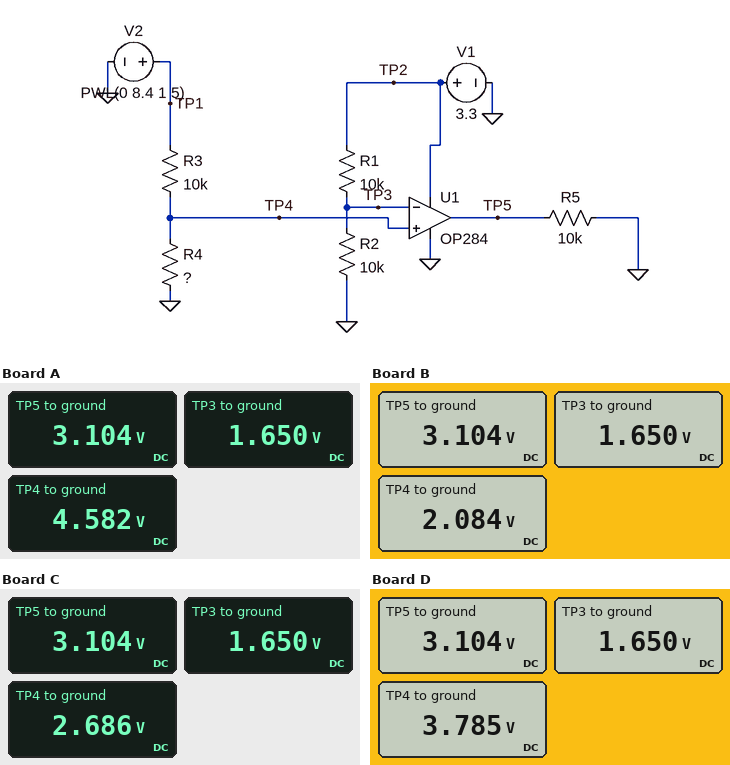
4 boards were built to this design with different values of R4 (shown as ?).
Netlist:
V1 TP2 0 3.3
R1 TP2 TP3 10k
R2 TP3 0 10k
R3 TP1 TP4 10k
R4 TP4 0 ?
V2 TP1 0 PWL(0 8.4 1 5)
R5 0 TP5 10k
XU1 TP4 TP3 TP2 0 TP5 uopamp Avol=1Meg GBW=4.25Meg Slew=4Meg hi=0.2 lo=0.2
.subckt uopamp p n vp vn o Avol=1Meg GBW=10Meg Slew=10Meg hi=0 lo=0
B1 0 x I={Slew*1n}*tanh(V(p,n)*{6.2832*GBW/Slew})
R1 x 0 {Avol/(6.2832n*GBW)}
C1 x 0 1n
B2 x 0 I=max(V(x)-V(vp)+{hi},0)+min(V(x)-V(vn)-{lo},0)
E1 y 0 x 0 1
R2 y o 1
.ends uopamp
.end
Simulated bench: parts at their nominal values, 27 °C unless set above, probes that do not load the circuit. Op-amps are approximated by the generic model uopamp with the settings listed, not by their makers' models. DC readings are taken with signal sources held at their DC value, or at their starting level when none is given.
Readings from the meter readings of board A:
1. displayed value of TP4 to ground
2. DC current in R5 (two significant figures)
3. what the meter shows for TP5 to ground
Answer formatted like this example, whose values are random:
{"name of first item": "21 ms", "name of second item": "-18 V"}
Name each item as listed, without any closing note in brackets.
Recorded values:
{"displayed value of TP4 to ground": "4.582 V", "DC current in R5": "310 µA", "what the meter shows for TP5 to ground": "3.104 V"}
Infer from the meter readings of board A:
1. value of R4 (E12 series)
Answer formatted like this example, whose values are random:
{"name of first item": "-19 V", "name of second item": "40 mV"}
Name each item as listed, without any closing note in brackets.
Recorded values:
{"value of R4": "12 kΩ"}
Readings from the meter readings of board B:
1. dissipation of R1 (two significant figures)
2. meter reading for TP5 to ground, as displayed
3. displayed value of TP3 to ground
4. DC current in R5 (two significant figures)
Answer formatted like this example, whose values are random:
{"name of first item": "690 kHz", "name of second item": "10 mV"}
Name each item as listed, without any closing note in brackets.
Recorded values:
{"dissipation of R1": "270 µW", "meter reading for TP5 to ground, as displayed": "3.104 V", "displayed value of TP3 to ground": "1.650 V", "DC current in R5": "310 µA"}
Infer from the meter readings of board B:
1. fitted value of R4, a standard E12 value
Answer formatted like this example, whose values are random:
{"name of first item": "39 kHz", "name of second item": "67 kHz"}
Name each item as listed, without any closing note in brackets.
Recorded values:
{"fitted value of R4, a standard E12 value": "3.3 kΩ"}
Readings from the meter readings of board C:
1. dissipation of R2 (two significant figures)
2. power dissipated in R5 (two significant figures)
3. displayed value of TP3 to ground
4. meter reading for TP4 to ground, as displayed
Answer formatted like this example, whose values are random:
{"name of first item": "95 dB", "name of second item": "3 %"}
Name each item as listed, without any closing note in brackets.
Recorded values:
{"dissipation of R2": "270 µW", "power dissipated in R5": "960 µW", "displayed value of TP3 to ground": "1.650 V", "meter reading for TP4 to ground, as displayed": "2.686 V"}
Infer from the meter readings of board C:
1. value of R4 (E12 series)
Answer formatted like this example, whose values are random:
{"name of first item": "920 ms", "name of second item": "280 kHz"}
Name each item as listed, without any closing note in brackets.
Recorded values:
{"value of R4": "4.7 kΩ"}
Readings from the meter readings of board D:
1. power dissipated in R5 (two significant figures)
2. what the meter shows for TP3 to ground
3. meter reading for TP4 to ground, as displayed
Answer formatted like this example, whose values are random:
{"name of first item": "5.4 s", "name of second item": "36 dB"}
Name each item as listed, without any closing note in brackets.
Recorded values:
{"power dissipated in R5": "960 µW", "what the meter shows for TP3 to ground": "1.650 V", "meter reading for TP4 to ground, as displayed": "3.785 V"}
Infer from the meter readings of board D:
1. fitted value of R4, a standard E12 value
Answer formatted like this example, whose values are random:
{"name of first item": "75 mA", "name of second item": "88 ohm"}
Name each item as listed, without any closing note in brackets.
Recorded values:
{"fitted value of R4, a standard E12 value": "8.2 kΩ"}
